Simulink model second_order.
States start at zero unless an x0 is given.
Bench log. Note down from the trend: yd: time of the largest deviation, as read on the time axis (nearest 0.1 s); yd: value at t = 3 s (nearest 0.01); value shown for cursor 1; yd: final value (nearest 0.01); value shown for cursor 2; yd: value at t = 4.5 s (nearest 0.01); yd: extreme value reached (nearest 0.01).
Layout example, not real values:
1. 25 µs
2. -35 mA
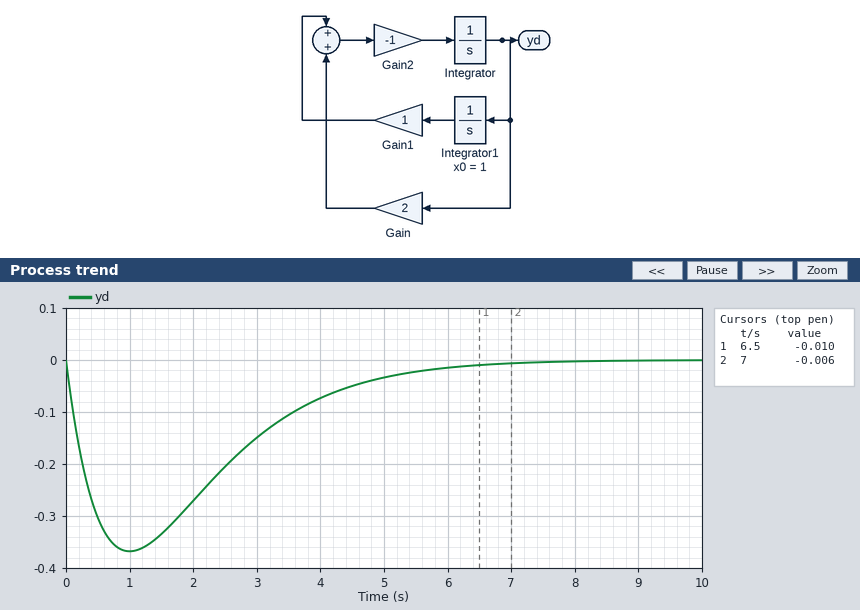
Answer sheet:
1. 1.0 s
2. -0.15
3. -0.010
4. 0.00
5. -0.006
6. -0.05
7. -0.37
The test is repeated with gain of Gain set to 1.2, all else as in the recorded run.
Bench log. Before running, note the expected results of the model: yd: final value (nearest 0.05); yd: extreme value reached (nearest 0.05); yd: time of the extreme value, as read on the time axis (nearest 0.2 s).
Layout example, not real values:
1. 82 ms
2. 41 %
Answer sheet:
1. 0.00
2. -0.50
3. 1.2 s
